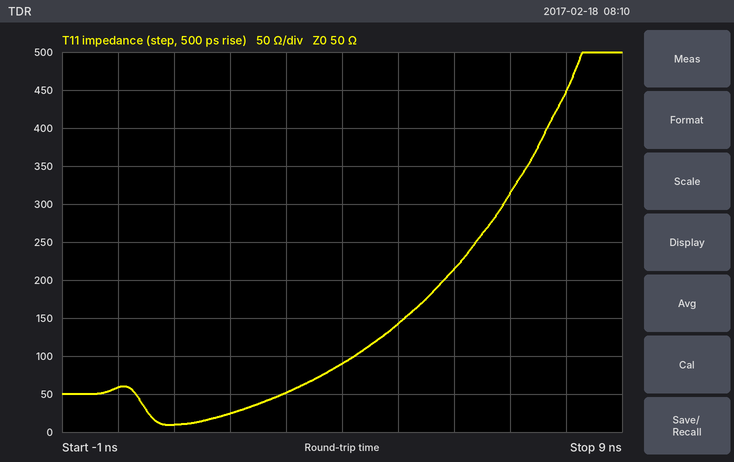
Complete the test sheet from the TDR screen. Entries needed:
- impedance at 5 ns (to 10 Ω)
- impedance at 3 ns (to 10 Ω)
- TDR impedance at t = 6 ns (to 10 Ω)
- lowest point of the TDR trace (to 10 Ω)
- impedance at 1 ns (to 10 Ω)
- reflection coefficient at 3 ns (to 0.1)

140 Ω
50 Ω
210 Ω
10 Ω
10 Ω
0.0
